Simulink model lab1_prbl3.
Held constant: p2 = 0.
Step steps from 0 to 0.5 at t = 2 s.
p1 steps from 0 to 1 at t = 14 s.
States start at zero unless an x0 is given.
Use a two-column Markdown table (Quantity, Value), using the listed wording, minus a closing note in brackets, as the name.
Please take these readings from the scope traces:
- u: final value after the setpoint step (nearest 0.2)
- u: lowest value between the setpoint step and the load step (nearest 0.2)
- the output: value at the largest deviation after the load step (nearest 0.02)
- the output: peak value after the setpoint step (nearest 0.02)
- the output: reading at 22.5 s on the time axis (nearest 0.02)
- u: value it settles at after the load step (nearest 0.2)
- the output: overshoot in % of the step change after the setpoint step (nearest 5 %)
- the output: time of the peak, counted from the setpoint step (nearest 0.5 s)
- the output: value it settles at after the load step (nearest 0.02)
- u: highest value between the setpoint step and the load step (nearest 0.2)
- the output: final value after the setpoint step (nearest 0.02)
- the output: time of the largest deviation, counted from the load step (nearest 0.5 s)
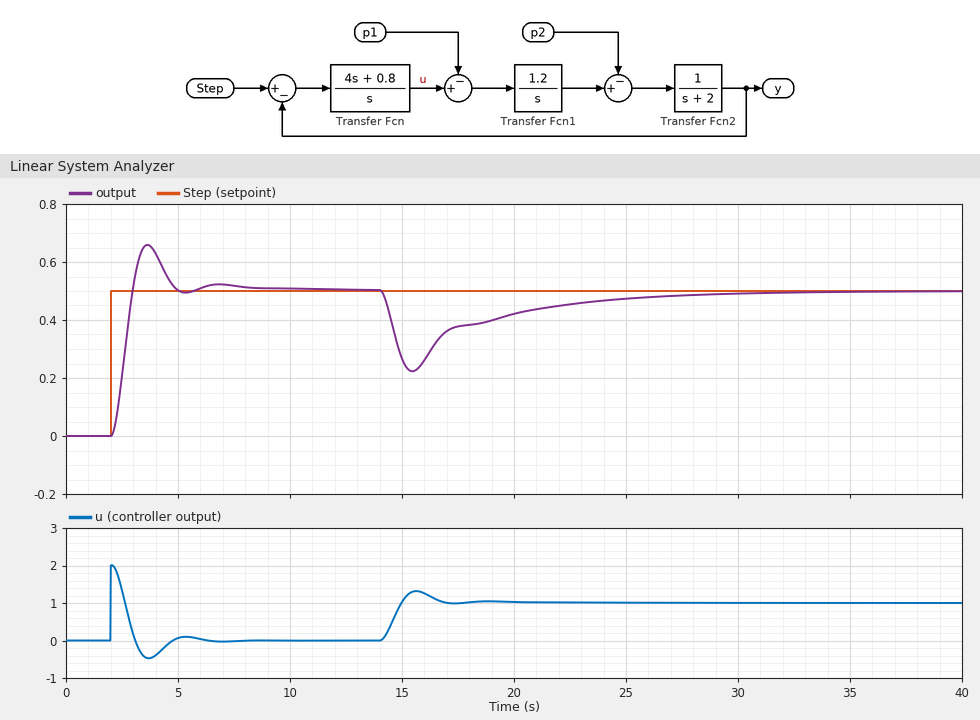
| Quantity | Value |
|---|---|
| u: final value after the setpoint step | 0.0 |
| u: lowest value between the setpoint step and the load step | -0.4 |
| the output: value at the largest deviation after the load step | 0.22 |
| the output: peak value after the setpoint step | 0.66 |
| the output: reading at 22.5 s on the time axis | 0.46 |
| u: value it settles at after the load step | 1.0 |
| the output: overshoot in % of the step change after the setpoint step | 30 % |
| the output: time of the peak, counted from the setpoint step | 1.5 s |
| the output: value it settles at after the load step | 0.50 |
| u: highest value between the setpoint step and the load step | 2.0 |
| the output: final value after the setpoint step | 0.50 |
| the output: time of the largest deviation, counted from the load step | 1.5 s |
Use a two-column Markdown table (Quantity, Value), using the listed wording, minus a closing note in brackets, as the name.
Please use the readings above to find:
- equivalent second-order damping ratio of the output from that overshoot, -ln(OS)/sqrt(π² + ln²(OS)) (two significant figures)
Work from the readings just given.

| Quantity | Value |
|---|---|
| equivalent second-order damping ratio of the output from that overshoot, -ln(OS)/sqrt(π² + ln²(OS)) | 0.36 |
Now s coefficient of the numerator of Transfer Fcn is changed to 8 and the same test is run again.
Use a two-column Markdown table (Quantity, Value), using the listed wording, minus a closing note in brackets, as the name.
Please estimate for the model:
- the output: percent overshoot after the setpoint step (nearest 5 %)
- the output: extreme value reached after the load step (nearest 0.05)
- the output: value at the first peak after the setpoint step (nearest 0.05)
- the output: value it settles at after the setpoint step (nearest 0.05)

| Quantity | Value |
|---|---|
| the output: percent overshoot after the setpoint step | 40 % |
| the output: extreme value reached after the load step | 0.35 |
| the output: value at the first peak after the setpoint step | 0.70 |
| the output: value it settles at after the setpoint step | 0.50 |
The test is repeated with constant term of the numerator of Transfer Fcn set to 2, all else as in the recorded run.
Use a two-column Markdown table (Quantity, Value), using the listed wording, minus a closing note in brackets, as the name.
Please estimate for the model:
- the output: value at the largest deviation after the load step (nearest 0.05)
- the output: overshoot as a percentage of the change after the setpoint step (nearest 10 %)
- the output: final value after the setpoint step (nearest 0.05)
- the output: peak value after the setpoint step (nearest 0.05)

| Quantity | Value |
|---|---|
| the output: value at the largest deviation after the load step | 0.25 |
| the output: overshoot as a percentage of the change after the setpoint step | 50 % |
| the output: final value after the setpoint step | 0.50 |
| the output: peak value after the setpoint step | 0.75 |
